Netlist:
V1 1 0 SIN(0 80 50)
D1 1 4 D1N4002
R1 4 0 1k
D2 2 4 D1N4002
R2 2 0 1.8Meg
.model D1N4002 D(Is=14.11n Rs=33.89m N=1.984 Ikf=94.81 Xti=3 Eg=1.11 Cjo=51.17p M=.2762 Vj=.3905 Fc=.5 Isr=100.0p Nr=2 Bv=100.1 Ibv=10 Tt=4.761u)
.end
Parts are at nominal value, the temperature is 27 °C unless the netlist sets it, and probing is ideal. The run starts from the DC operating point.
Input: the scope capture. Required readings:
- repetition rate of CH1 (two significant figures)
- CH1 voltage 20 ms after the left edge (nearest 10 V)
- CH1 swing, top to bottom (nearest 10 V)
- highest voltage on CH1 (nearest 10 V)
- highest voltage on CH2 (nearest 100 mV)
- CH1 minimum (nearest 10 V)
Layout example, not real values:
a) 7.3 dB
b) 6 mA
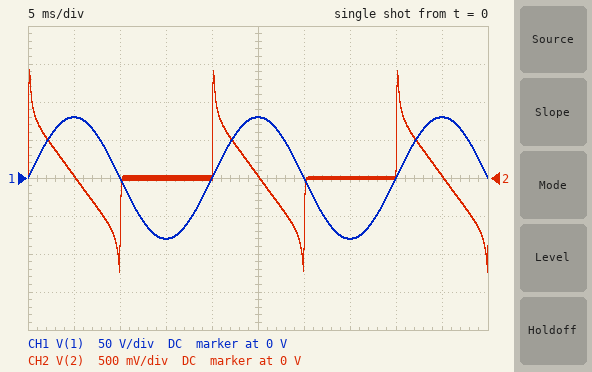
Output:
a) 50 Hz
b) 0 V
c) 160 V
d) 80 V
e) 1.4 V
f) -80 V
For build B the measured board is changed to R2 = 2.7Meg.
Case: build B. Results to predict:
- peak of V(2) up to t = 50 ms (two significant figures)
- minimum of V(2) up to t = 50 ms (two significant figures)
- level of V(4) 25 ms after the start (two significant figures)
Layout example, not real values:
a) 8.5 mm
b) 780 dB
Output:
a) 2.0 V
b) -1.7 V
c) 79 V
